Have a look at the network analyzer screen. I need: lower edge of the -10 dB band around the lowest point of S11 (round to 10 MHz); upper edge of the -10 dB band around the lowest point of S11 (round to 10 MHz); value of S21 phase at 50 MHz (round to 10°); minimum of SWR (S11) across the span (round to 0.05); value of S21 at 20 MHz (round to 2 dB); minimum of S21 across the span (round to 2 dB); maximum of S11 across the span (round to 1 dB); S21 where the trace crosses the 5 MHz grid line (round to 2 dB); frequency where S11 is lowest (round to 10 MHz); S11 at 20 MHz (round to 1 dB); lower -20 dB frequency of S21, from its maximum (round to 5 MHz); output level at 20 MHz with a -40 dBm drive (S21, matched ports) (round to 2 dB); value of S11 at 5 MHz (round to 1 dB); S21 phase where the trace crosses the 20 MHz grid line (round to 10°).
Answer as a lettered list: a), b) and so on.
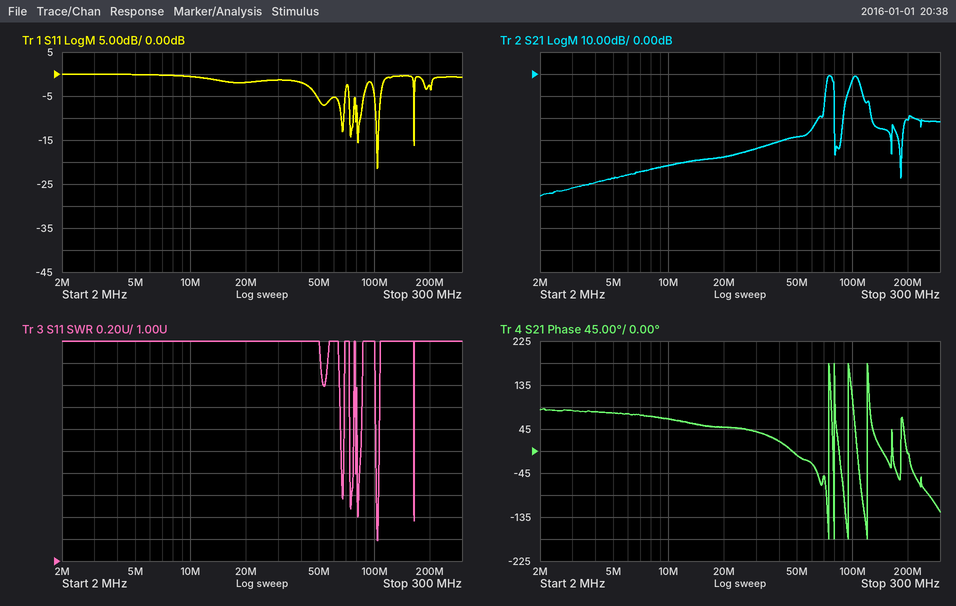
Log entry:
a) 100 MHz
b) 110 MHz
c) -10°
d) 1.20
e) -38 dB
f) -56 dB
g) 0 dB
h) -48 dB
i) 100 MHz
j) -2 dB
k) 65 MHz
l) -78 dBm
m) 0 dB
n) 50°
